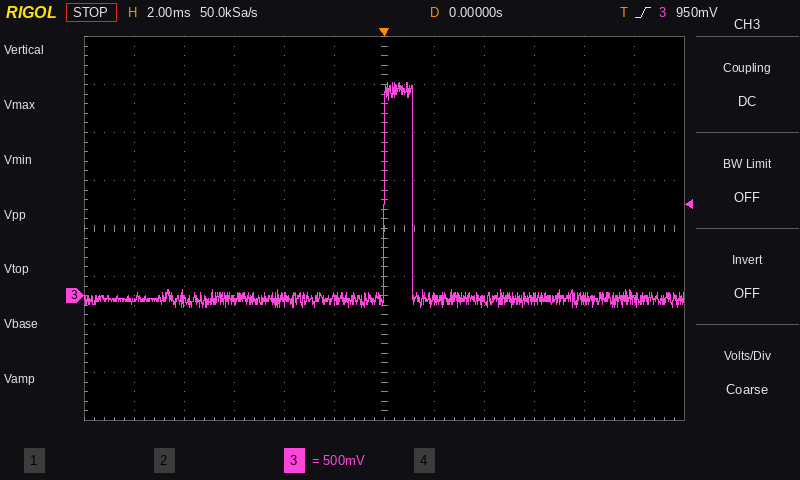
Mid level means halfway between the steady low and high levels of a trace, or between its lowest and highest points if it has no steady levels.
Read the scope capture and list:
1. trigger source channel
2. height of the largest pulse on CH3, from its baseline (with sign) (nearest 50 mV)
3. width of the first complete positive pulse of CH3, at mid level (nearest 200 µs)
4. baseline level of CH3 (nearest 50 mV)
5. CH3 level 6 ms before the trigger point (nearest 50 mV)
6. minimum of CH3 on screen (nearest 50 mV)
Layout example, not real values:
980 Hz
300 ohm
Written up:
CH3
+2.25 V
1.2 ms
-50 mV
-50 mV
-100 mV
